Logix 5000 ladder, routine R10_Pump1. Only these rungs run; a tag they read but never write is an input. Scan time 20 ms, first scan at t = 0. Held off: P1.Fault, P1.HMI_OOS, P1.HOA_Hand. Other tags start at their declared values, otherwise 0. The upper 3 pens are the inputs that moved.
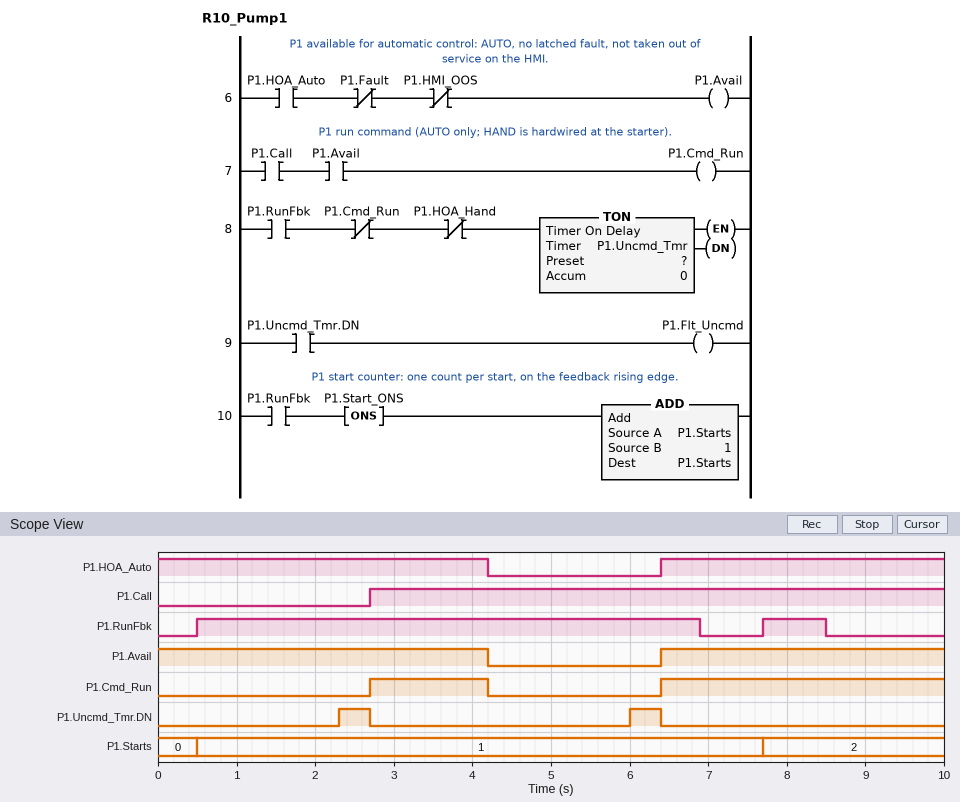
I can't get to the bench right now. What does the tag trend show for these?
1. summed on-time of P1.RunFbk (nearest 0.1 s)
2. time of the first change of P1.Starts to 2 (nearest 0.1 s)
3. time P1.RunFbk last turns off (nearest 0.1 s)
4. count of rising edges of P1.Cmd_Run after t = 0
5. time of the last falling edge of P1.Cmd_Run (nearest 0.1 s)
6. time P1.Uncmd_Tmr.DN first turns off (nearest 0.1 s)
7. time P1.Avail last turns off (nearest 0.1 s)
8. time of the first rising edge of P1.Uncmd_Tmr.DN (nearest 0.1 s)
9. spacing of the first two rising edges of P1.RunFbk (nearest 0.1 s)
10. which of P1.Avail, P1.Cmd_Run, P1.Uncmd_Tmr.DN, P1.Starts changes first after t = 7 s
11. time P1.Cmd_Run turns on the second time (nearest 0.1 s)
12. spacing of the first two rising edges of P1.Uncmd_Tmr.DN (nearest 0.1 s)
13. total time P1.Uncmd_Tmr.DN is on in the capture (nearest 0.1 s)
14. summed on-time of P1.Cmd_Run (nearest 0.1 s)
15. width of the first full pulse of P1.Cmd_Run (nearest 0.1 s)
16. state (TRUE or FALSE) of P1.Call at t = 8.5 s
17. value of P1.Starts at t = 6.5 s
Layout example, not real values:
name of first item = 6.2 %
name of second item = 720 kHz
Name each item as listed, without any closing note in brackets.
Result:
summed on-time of P1.RunFbk = 7.2 s
time of the first change of P1.Starts to 2 = 7.7 s
time P1.RunFbk last turns off = 8.5 s
count of rising edges of P1.Cmd_Run after t = 0 = 2
time of the last falling edge of P1.Cmd_Run = 4.2 s
time P1.Uncmd_Tmr.DN first turns off = 2.7 s
time P1.Avail last turns off = 4.2 s
time of the first rising edge of P1.Uncmd_Tmr.DN = 2.3 s
spacing of the first two rising edges of P1.RunFbk = 7.2 s
which of P1.Avail, P1.Cmd_Run, P1.Uncmd_Tmr.DN, P1.Starts changes first after t = 7 s = P1.Starts
time P1.Cmd_Run turns on the second time = 6.4 s
spacing of the first two rising edges of P1.Uncmd_Tmr.DN = 3.7 s
total time P1.Uncmd_Tmr.DN is on in the capture = 0.8 s
summed on-time of P1.Cmd_Run = 5.1 s
width of the first full pulse of P1.Cmd_Run = 1.5 s
state (TRUE or FALSE) of P1.Call at t = 8.5 s = TRUE
value of P1.Starts at t = 6.5 s = 1
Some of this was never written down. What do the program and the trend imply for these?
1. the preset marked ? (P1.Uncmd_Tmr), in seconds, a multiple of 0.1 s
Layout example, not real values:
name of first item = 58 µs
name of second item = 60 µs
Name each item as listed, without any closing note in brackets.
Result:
the preset marked ? (P1.Uncmd_Tmr), in seconds, a multiple of 0.1 s = 1.8 s
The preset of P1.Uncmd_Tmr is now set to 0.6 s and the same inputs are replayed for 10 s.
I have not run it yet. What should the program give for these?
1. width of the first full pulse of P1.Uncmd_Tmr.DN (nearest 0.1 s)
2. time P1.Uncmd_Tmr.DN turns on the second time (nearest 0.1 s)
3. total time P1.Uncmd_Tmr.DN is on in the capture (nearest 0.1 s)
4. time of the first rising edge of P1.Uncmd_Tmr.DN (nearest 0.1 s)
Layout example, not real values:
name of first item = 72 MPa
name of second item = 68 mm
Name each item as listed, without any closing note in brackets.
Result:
width of the first full pulse of P1.Uncmd_Tmr.DN = 1.6 s
time P1.Uncmd_Tmr.DN turns on the second time = 4.8 s
total time P1.Uncmd_Tmr.DN is on in the capture = 3.2 s
time of the first rising edge of P1.Uncmd_Tmr.DN = 1.1 s
